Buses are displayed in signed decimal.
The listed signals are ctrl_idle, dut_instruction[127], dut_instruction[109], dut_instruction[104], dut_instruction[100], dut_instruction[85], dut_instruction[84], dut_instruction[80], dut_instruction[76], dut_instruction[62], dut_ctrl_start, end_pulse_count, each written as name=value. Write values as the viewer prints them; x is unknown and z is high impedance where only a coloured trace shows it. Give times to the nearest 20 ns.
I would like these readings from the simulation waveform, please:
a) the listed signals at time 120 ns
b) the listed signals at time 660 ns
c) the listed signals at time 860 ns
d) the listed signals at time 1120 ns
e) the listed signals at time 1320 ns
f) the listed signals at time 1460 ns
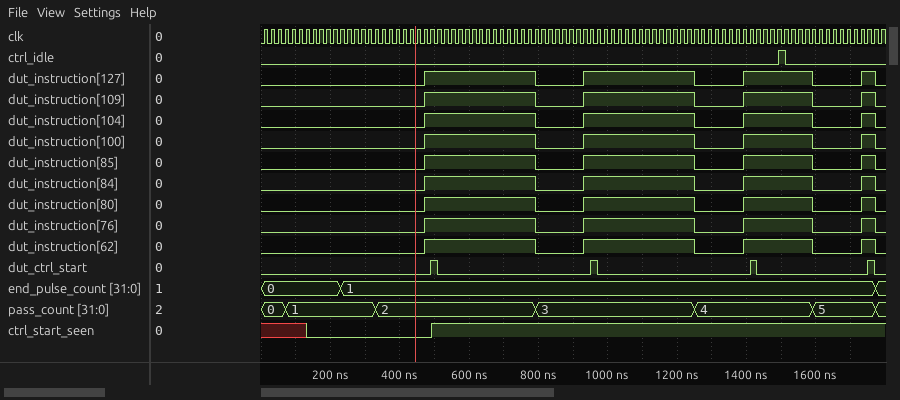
ctrl_idle=0, dut_instruction[127]=0, dut_instruction[109]=0, dut_instruction[104]=0, dut_instruction[100]=0, dut_instruction[85]=0, dut_instruction[84]=0, dut_instruction[80]=0, dut_instruction[76]=0, dut_instruction[62]=0, dut_ctrl_start=0, end_pulse_count=0
ctrl_idle=0, dut_instruction[127]=1, dut_instruction[109]=1, dut_instruction[104]=1, dut_instruction[100]=1, dut_instruction[85]=1, dut_instruction[84]=1, dut_instruction[80]=1, dut_instruction[76]=1, dut_instruction[62]=1, dut_ctrl_start=0, end_pulse_count=1
ctrl_idle=0, dut_instruction[127]=0, dut_instruction[109]=0, dut_instruction[104]=0, dut_instruction[100]=0, dut_instruction[85]=0, dut_instruction[84]=0, dut_instruction[80]=0, dut_instruction[76]=0, dut_instruction[62]=0, dut_ctrl_start=0, end_pulse_count=1
ctrl_idle=0, dut_instruction[127]=1, dut_instruction[109]=1, dut_instruction[104]=1, dut_instruction[100]=1, dut_instruction[85]=1, dut_instruction[84]=1, dut_instruction[80]=1, dut_instruction[76]=1, dut_instruction[62]=1, dut_ctrl_start=0, end_pulse_count=1
ctrl_idle=0, dut_instruction[127]=0, dut_instruction[109]=0, dut_instruction[104]=0, dut_instruction[100]=0, dut_instruction[85]=0, dut_instruction[84]=0, dut_instruction[80]=0, dut_instruction[76]=0, dut_instruction[62]=0, dut_ctrl_start=0, end_pulse_count=1
ctrl_idle=0, dut_instruction[127]=1, dut_instruction[109]=1, dut_instruction[104]=1, dut_instruction[100]=1, dut_instruction[85]=1, dut_instruction[84]=1, dut_instruction[80]=1, dut_instruction[76]=1, dut_instruction[62]=1, dut_ctrl_start=0, end_pulse_count=1
